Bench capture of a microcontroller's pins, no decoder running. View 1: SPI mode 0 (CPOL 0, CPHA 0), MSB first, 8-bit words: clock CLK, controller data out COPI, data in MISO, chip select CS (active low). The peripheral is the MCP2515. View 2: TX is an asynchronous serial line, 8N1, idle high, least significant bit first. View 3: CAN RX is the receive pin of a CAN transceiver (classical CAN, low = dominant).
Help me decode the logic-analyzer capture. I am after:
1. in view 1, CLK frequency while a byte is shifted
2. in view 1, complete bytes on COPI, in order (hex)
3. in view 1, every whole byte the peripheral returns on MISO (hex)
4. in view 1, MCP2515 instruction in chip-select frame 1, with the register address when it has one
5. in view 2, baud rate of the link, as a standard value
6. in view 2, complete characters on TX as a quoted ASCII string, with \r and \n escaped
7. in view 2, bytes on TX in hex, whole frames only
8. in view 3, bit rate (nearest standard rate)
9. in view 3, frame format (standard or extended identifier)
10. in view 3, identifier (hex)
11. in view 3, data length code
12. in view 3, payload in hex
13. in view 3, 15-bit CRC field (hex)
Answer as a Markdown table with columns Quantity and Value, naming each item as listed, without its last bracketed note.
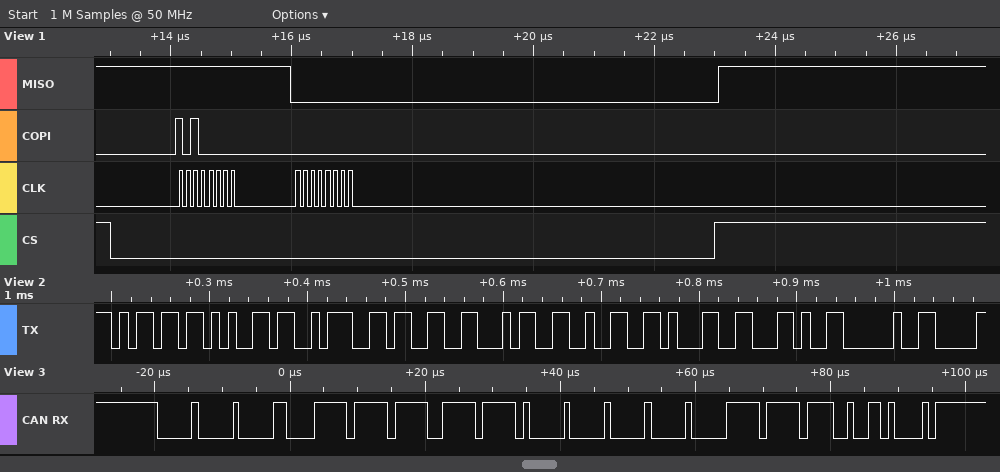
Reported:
| Quantity | Value |
|---|---|
| in view 1, CLK frequency while a byte is shifted | 8 MHz |
| in view 1, complete bytes on COPI, in order | A0 00 |
| in view 1, every whole byte the peripheral returns on MISO | FF 00 |
| in view 1, MCP2515 instruction in chip-select frame 1, with the register address when it has one | READ STATUS |
| in view 2, baud rate of the link, as a standard value | 115200 baud |
| in view 2, complete characters on TX as a quoted ASCII string, with \r and \n escaped | "me:3421, " |
| in view 2, bytes on TX in hex, whole frames only | 6D 65 3A 33 34 32 31 2C 20 |
| in view 3, bit rate | 1000 kbit/s |
| in view 3, frame format | standard |
| in view 3, identifier | 0x000 |
| in view 3, data length code | 8 |
| in view 3, payload in hex | 7F FF 7F F0 00 00 07 FF |
| in view 3, 15-bit CRC field | 0x64D0 |
